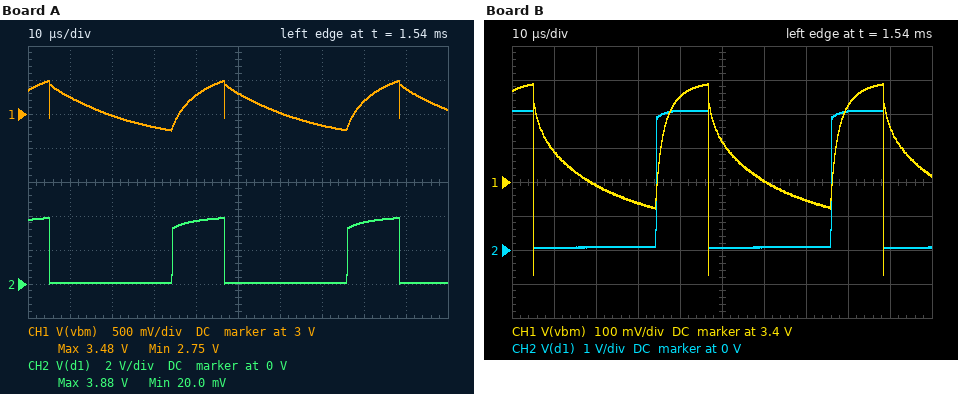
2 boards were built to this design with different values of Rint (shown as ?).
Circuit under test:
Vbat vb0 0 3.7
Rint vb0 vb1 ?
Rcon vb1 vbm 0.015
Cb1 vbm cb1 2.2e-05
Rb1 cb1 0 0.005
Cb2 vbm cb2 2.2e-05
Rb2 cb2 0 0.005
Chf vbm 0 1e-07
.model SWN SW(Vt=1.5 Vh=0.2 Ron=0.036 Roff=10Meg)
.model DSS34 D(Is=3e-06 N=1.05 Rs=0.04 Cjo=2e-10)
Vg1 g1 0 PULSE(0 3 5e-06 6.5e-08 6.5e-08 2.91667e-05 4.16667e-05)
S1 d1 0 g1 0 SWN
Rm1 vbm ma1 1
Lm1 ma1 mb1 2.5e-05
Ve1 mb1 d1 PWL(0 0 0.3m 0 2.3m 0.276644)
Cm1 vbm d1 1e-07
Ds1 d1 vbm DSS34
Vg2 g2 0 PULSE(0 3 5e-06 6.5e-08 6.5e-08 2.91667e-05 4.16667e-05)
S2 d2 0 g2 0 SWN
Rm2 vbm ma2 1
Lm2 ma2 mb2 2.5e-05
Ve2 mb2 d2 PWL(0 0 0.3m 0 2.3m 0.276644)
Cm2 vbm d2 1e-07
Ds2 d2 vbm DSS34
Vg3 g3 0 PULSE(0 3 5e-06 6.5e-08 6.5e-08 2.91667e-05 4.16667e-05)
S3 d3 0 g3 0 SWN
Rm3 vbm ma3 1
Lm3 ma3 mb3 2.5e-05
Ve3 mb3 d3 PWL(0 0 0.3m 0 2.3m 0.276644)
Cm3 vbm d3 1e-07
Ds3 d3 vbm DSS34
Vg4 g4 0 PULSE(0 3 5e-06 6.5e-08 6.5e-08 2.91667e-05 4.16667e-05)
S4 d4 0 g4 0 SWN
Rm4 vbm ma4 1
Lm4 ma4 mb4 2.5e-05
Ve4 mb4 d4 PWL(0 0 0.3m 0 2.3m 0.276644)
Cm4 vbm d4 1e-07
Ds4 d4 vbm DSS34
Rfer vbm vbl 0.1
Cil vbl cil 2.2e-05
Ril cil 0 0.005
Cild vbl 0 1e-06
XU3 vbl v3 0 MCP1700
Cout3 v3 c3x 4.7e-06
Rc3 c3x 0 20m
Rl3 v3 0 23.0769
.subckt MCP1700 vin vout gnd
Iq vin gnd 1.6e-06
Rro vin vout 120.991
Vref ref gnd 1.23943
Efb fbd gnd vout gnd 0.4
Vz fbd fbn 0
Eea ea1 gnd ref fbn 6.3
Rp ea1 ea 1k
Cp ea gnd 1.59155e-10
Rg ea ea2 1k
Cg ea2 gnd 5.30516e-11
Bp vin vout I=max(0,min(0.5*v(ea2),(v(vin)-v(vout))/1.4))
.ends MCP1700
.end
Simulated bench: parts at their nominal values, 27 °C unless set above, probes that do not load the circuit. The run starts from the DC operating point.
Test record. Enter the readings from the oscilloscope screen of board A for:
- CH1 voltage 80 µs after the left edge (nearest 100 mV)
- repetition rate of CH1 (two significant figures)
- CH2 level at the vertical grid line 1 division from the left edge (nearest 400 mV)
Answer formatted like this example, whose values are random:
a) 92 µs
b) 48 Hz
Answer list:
a) 3.2 V
b) 24 kHz
c) 0 V
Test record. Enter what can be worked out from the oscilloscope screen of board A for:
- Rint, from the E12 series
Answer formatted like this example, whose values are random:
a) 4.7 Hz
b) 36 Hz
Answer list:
a) 0.1 Ω
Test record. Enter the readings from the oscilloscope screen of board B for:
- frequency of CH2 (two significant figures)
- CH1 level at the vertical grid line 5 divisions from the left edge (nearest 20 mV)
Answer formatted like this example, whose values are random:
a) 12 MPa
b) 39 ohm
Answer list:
a) 24 kHz
b) 3.52 V
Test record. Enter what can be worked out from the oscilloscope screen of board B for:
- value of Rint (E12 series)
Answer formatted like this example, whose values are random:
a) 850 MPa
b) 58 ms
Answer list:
a) 0.022 Ω
